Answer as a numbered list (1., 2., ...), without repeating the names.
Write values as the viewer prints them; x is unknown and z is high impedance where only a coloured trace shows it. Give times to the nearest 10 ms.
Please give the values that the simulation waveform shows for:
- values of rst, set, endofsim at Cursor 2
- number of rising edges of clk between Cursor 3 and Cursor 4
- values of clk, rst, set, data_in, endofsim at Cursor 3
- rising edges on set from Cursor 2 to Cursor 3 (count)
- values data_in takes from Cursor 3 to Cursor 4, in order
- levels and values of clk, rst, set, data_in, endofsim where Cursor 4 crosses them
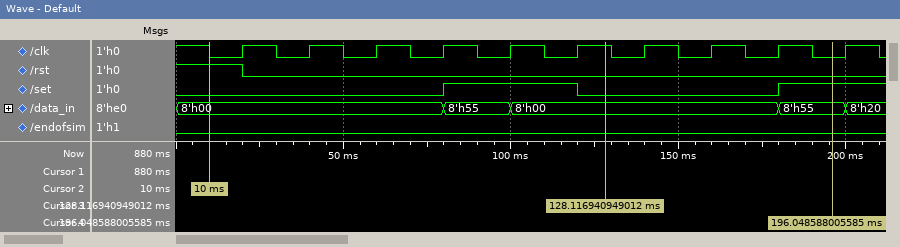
1. rst=1, set=0, endofsim=0
2. 3
3. clk=1, rst=0, set=0, data_in=8'h00, endofsim=0
4. 1
5. 8'h00, 8'h55
6. clk=0, rst=0, set=1, data_in=8'h55, endofsim=0
